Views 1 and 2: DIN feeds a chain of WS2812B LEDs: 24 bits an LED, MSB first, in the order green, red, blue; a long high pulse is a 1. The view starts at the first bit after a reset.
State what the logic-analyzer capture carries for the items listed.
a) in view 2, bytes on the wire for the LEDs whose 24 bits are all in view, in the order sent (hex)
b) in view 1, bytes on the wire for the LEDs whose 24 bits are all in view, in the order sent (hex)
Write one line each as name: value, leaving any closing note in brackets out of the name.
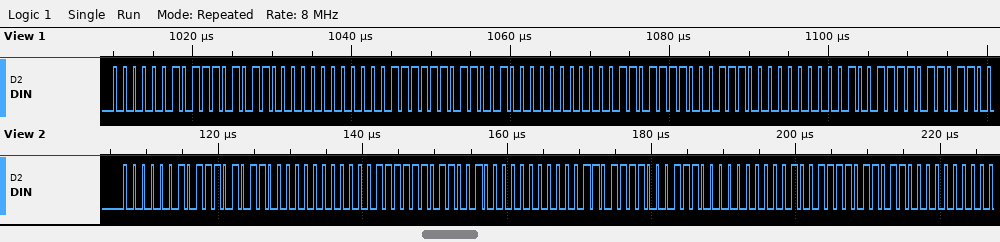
in view 2, bytes on the wire for the LEDs whose 24 bits are all in view, in the order sent: 02 EB 00 0F D9 00 1B C7 00 27 B6 00
in view 1, bytes on the wire for the LEDs whose 24 bits are all in view, in the order sent: 02 EB 00 0F D9 00 1B C7 00
